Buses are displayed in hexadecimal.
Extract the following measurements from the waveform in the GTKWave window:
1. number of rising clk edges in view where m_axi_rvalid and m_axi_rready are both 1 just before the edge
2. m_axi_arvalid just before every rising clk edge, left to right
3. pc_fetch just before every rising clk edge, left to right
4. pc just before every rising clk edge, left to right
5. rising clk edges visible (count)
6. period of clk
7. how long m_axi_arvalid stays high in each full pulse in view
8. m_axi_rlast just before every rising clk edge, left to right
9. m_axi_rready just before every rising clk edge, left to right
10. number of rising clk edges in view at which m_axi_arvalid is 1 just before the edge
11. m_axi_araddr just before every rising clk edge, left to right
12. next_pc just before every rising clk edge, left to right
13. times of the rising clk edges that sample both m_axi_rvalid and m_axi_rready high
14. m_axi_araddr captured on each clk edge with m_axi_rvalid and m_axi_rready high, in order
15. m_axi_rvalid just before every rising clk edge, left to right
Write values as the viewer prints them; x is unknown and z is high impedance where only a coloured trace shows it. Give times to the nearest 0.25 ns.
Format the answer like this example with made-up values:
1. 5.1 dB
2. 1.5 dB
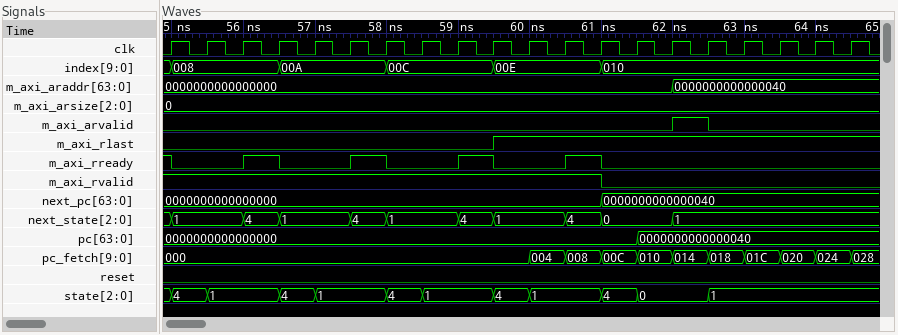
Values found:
1. 5
2. 0 0 0 0 0 0 0 0 0 0 0 0 0 0 0 1 0 0 0 0
3. 000, 000, 000, 000, 000, 000, 000, 000, 000, 000, 000, 004, 008, 00C, 010, 014, 018, 01C, 020, 024
4. 0000000000000000, 0000000000000000, 0000000000000000, 0000000000000000, 0000000000000000, 0000000000000000, 0000000000000000, 0000000000000000, 0000000000000000, 0000000000000000, 0000000000000000, 0000000000000000, 0000000000000000, 0000000000000000, 0000000000000040, 0000000000000040, 0000000000000040, 0000000000000040, 0000000000000040, 0000000000000040
5. 20
6. 0.5 ns
7. 0.5 ns
8. 0 0 0 0 0 0 0 0 0 0 1 1 1 1 1 1 1 1 1 1
9. 1 0 0 1 0 0 1 0 0 1 0 0 1 0 0 0 0 0 0 0
10. 1
11. 0000000000000000, 0000000000000000, 0000000000000000, 0000000000000000, 0000000000000000, 0000000000000000, 0000000000000000, 0000000000000000, 0000000000000000, 0000000000000000, 0000000000000000, 0000000000000000, 0000000000000000, 0000000000000000, 0000000000000000, 0000000000000040, 0000000000000040, 0000000000000040, 0000000000000040, 0000000000000040
12. 0000000000000000, 0000000000000000, 0000000000000000, 0000000000000000, 0000000000000000, 0000000000000000, 0000000000000000, 0000000000000000, 0000000000000000, 0000000000000000, 0000000000000000, 0000000000000000, 0000000000000000, 0000000000000040, 0000000000000040, 0000000000000040, 0000000000000040, 0000000000000040, 0000000000000040, 0000000000000040
13. 55 ns, 56.5 ns, 58 ns, 59.5 ns, 61 ns
14. 0000000000000000, 0000000000000000, 0000000000000000, 0000000000000000, 0000000000000000
15. 1 1 1 1 1 1 1 1 1 1 1 1 1 0 0 0 0 0 0 0
